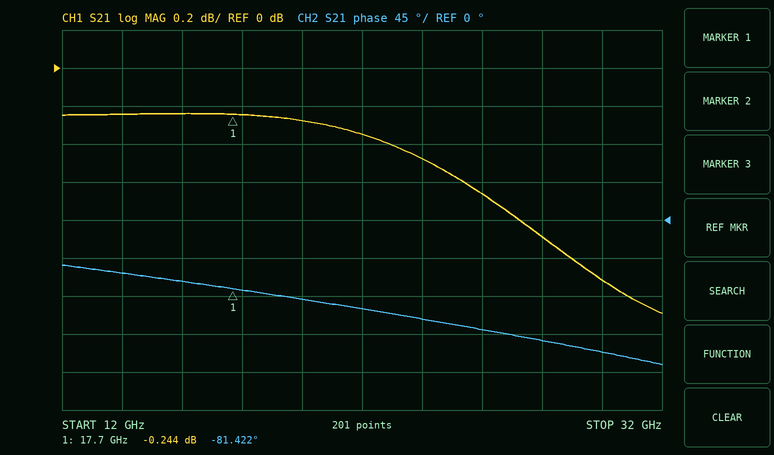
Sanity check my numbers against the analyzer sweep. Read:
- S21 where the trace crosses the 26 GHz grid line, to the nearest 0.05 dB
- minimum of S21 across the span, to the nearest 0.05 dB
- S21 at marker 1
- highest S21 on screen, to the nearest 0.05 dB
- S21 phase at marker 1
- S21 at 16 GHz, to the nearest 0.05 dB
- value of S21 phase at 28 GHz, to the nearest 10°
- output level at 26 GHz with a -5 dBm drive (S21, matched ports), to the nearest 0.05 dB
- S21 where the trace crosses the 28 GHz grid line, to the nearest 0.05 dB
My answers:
-0.65 dB
-1.30 dB
-0.244 dB
-0.25 dB
-81.422°
-0.25 dB
-140°
-5.65 dBm
-0.90 dB
